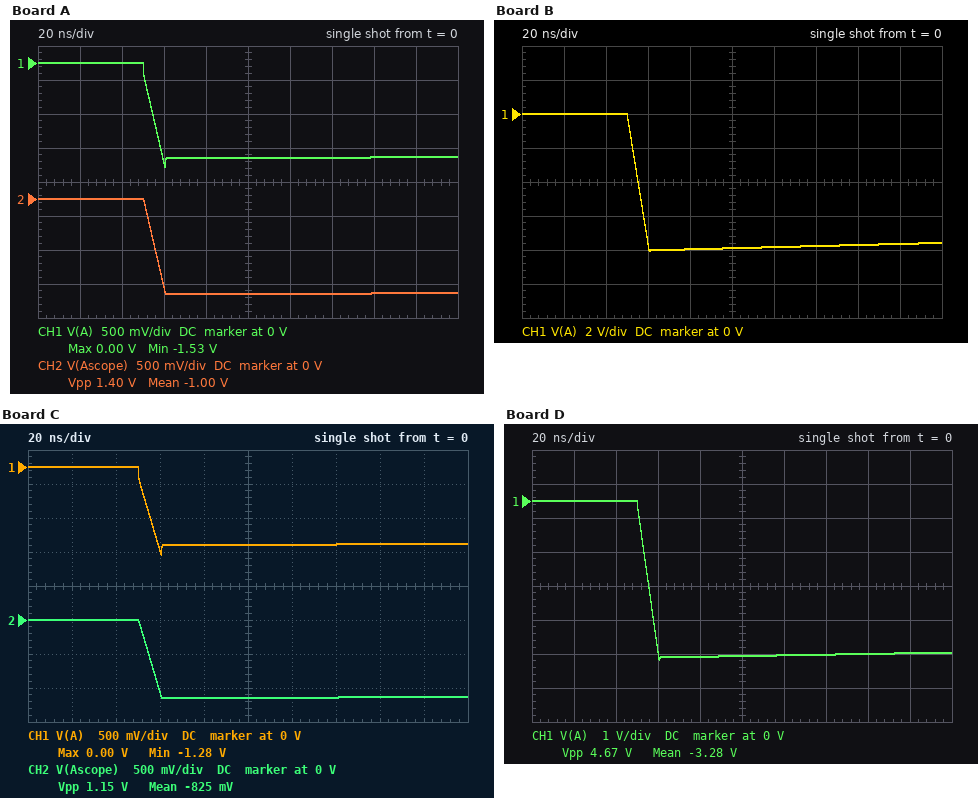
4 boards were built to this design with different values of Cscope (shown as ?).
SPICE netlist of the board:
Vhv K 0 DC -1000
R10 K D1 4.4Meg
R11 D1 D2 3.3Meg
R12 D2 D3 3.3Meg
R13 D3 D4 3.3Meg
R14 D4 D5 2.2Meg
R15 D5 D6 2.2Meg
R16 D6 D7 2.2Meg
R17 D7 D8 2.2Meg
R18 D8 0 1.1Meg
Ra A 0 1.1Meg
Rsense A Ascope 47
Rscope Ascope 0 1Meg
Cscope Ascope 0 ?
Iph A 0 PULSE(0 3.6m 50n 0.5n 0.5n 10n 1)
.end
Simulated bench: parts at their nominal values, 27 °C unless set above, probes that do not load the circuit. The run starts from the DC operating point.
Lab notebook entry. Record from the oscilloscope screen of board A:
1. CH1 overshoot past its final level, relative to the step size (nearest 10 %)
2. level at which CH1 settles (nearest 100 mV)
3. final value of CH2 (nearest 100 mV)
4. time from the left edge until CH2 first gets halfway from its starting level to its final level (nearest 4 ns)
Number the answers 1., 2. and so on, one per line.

1. 10 %
2. -1.4 V
3. -1.4 V
4. 56 ns
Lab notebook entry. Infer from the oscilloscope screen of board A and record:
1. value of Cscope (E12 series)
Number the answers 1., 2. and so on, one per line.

1. 27 pF
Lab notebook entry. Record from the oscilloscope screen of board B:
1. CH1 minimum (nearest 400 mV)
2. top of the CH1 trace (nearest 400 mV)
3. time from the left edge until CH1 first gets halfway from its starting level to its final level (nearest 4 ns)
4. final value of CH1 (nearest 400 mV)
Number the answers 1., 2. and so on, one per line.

1. -8.0 V
2. 0 V
3. 56 ns
4. -7.6 V
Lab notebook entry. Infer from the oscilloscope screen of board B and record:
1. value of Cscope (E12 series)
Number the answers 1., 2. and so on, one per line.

1. 4.7 pF
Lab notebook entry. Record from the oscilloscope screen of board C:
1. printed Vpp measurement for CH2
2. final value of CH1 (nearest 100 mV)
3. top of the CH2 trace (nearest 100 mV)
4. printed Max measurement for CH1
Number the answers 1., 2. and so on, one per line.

1. 1.15 V
2. -1.1 V
3. 0 V
4. 0.00 V
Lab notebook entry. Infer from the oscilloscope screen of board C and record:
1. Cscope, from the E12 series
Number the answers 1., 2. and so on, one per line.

1. 33 pF
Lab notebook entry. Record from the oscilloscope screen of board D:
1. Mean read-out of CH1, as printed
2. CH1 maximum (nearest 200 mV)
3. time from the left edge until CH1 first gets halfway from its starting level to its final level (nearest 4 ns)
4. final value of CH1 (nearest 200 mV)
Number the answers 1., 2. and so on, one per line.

1. -3.28 V
2. 0 V
3. 56 ns
4. -4.4 V
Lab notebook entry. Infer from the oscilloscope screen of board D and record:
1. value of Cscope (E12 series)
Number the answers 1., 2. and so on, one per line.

1. 8.2 pF
